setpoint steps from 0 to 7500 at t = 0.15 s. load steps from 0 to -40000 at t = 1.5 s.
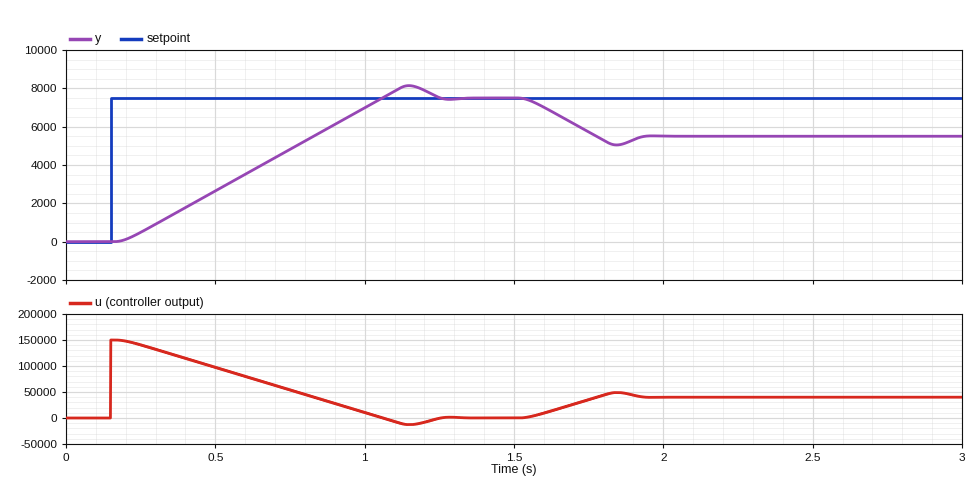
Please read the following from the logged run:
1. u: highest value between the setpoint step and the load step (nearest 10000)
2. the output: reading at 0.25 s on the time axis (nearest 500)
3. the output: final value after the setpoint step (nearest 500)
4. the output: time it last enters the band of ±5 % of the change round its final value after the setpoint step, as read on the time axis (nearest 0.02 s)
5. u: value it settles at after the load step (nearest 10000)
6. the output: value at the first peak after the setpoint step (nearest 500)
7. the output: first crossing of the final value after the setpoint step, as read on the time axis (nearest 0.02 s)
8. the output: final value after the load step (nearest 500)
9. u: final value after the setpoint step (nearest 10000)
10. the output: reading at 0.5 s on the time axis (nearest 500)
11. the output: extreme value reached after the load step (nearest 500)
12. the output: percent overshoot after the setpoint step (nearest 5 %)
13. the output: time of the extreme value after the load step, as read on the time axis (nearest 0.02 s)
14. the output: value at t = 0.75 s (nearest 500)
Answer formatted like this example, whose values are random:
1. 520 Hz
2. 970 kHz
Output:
1. 150000
2. 500
3. 7500
4. 1.20 s
5. 40000
6. 8000
7. 1.06 s
8. 5500
9. 0
10. 2500
11. 5000
12. 10 %
13. 1.84 s
14. 5000
